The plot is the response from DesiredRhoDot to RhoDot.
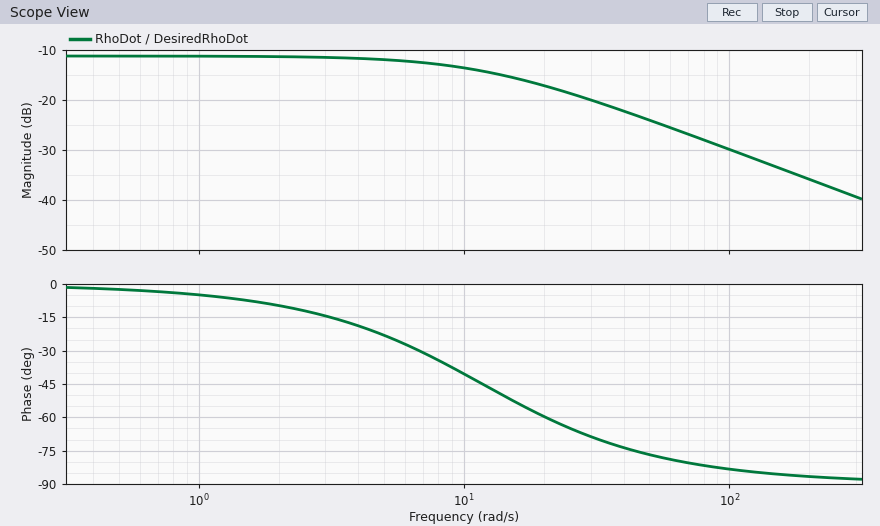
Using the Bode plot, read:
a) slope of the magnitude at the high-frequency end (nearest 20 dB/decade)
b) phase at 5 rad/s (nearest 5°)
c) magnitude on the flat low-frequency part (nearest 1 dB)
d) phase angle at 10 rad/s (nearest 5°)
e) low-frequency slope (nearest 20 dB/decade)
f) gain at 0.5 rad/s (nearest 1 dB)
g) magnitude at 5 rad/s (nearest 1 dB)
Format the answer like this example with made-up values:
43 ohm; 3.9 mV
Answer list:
-20 dB/decade; -25°; -11 dB; -40°; 0 dB/decade; -11 dB; -12 dB
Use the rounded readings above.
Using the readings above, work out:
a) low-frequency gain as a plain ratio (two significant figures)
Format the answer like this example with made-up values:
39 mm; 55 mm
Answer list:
0.28
